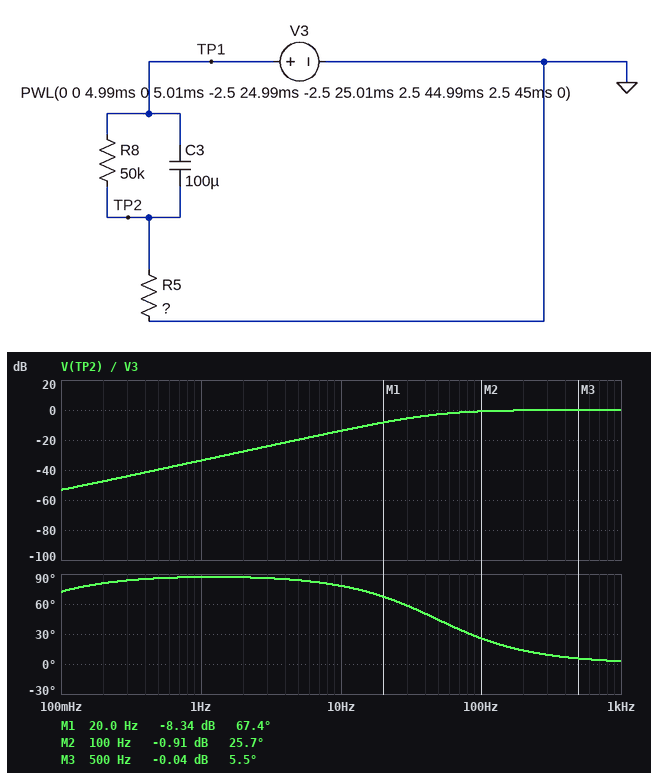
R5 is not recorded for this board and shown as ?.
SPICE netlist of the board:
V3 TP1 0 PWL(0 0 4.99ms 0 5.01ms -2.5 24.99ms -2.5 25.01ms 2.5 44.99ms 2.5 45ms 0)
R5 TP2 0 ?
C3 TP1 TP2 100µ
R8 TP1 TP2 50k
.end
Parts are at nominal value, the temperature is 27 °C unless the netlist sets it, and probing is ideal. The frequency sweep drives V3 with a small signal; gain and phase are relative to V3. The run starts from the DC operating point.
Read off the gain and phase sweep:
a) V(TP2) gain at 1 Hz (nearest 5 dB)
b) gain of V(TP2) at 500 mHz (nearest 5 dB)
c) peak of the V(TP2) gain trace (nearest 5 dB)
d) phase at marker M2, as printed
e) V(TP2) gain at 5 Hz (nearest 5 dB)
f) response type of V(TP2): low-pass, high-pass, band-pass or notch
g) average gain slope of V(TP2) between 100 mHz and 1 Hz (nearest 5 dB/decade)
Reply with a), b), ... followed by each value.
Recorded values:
a) -35 dB
b) -40 dB
c) 0 dB
d) 25.7 deg
e) -20 dB
f) high-pass
g) 20 dB/decade
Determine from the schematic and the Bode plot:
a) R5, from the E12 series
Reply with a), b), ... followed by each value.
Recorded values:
a) 33 Ω
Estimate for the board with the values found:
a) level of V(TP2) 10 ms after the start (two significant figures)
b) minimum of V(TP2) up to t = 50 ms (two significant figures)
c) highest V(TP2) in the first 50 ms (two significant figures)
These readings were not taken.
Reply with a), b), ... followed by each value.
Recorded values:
a) -550 mV
b) -2.5 V
c) 5.0 V
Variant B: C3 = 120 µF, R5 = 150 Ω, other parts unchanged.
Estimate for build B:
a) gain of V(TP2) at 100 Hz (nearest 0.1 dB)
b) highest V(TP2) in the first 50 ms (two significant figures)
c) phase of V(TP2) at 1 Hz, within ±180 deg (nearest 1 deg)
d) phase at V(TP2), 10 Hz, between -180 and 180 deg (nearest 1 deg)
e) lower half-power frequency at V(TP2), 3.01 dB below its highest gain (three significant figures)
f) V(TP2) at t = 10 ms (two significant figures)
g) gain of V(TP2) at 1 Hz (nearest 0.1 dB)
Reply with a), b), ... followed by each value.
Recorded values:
a) 0 dB
b) 4.2 V
c) 82 deg
d) 41 deg
e) 8.87 Hz
f) -1.9 V
g) -19.0 dB
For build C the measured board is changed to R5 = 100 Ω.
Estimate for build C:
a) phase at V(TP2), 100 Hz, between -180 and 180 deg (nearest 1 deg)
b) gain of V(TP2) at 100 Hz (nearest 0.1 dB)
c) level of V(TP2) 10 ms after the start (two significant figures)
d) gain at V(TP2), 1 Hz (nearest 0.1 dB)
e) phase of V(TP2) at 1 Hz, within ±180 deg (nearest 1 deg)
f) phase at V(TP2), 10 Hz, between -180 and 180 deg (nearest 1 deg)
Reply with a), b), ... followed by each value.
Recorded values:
a) 9 deg
b) -0.1 dB
c) -1.5 V
d) -24.1 dB
e) 85 deg
f) 58 deg
